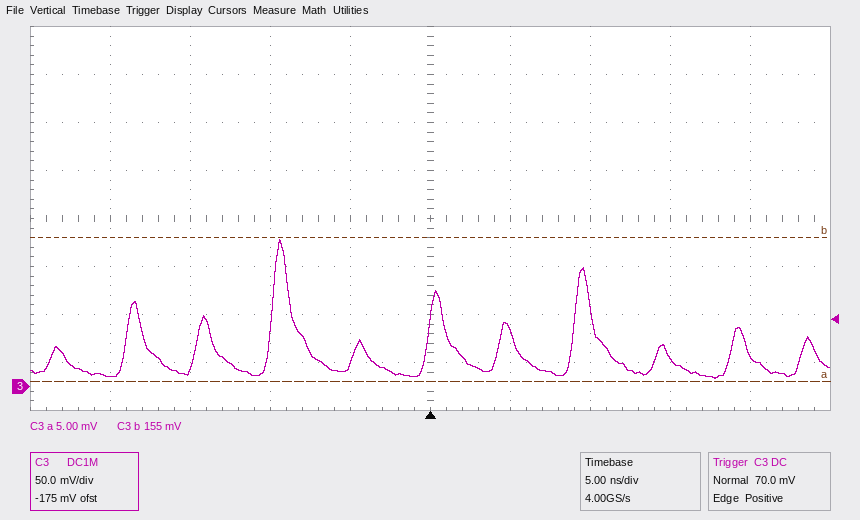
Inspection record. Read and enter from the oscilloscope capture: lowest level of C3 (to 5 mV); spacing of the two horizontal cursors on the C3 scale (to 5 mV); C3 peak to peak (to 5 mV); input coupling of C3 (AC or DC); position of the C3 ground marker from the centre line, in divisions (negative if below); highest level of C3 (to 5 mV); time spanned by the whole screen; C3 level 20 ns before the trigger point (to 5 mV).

10 mV
150 mV
145 mV
DC
-3.5 div
155 mV
50 ns
10 mV
